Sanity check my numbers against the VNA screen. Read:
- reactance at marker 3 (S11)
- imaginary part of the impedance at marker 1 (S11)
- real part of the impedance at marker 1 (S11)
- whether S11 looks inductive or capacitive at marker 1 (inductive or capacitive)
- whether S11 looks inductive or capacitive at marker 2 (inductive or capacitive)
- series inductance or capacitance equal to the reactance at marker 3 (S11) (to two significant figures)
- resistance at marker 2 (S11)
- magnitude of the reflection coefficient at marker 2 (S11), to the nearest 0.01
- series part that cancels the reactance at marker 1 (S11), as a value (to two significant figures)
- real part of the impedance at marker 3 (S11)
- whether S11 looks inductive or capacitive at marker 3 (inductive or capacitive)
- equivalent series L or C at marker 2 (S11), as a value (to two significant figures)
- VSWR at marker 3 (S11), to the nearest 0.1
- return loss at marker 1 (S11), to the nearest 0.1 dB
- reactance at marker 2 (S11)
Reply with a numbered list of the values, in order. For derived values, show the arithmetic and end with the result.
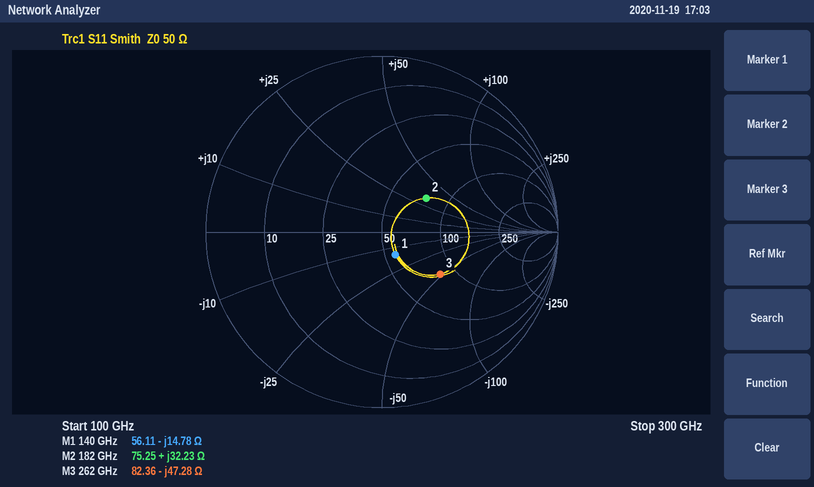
1. -47.28 Ω
2. -14.78 Ω
3. 56.11 Ω
4. capacitive
5. inductive
6. C = 1/(2π × 262 GHz × 47.28 Ω) ≈ 13 fF
7. 75.25 Ω
8. 0.32
9. L = 14.78 Ω/(2π × 140 GHz) ≈ 17 pH
10. 82.36 Ω
11. capacitive
12. L = 32.23 Ω/(2π × 182 GHz) ≈ 28 pH
13. 2.4
14. 16.5 dB
15. +32.23 Ω
